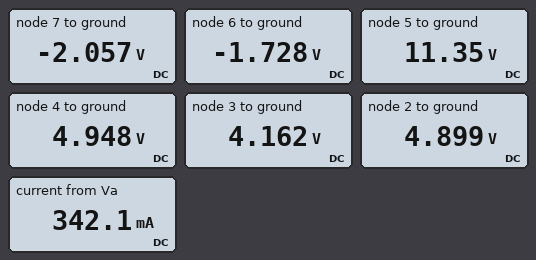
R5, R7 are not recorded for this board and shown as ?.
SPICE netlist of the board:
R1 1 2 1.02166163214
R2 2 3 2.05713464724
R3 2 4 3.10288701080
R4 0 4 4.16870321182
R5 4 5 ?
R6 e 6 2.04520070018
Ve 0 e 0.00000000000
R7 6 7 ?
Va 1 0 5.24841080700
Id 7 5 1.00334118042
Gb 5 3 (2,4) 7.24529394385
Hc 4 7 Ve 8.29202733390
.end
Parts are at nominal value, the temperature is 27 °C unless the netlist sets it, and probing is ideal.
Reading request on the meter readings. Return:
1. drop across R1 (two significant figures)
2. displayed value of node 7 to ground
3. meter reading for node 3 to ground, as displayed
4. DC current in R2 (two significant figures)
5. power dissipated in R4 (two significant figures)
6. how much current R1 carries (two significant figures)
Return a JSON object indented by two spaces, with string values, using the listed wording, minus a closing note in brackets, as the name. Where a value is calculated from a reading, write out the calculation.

{
  "drop across R1": "5.248 V - 4.899 V = 350 mV",
  "displayed value of node 7 to ground": "-2.057 V",
  "meter reading for node 3 to ground, as displayed": "4.162 V",
  "DC current in R2": "(4.899 V - 4.162 V) / 2.057 Ω = 360 mA",
  "power dissipated in R4": "(4.948 V)^2 / 4.169 Ω = 5.9 W",
  "how much current R1 carries": "(5.248 V - 4.899 V) / 1.022 Ω = 340 mA"
}
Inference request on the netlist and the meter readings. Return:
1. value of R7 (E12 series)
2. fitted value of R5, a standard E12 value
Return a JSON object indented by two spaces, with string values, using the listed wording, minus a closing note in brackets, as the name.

{
  "value of R7": "0.39 Ω",
  "fitted value of R5, a standard E12 value": "4.7 Ω"
}
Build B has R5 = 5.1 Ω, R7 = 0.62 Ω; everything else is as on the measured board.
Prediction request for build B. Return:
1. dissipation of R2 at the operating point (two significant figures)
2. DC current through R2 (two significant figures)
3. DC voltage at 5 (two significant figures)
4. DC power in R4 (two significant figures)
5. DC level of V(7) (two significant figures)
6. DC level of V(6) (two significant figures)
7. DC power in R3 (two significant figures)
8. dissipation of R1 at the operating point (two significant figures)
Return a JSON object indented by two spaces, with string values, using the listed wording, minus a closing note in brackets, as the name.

{
  "dissipation of R2 at the operating point": "220 mW",
  "DC current through R2": "320 mA",
  "DC voltage at 5": "12 V",
  "DC power in R4": "5.9 W",
  "DC level of V(7)": "-2.4 V",
  "DC level of V(6)": "-1.8 V",
  "DC power in R3": "640 µW",
  "dissipation of R1 at the operating point": "98 mW"
}
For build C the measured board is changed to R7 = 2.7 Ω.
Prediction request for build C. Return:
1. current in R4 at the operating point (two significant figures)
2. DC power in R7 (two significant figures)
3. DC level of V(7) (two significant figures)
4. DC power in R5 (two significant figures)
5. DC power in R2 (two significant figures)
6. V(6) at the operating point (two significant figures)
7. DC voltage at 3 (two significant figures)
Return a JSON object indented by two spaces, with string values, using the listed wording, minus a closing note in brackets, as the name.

{
  "current in R4 at the operating point": "1.3 A",
  "DC power in R7": "6.4 W",
  "DC level of V(7)": "-7.3 V",
  "DC power in R5": "2.7 W",
  "DC power in R2": "120 mW",
  "V(6) at the operating point": "-3.1 V",
  "DC voltage at 3": "6.0 V"
}
